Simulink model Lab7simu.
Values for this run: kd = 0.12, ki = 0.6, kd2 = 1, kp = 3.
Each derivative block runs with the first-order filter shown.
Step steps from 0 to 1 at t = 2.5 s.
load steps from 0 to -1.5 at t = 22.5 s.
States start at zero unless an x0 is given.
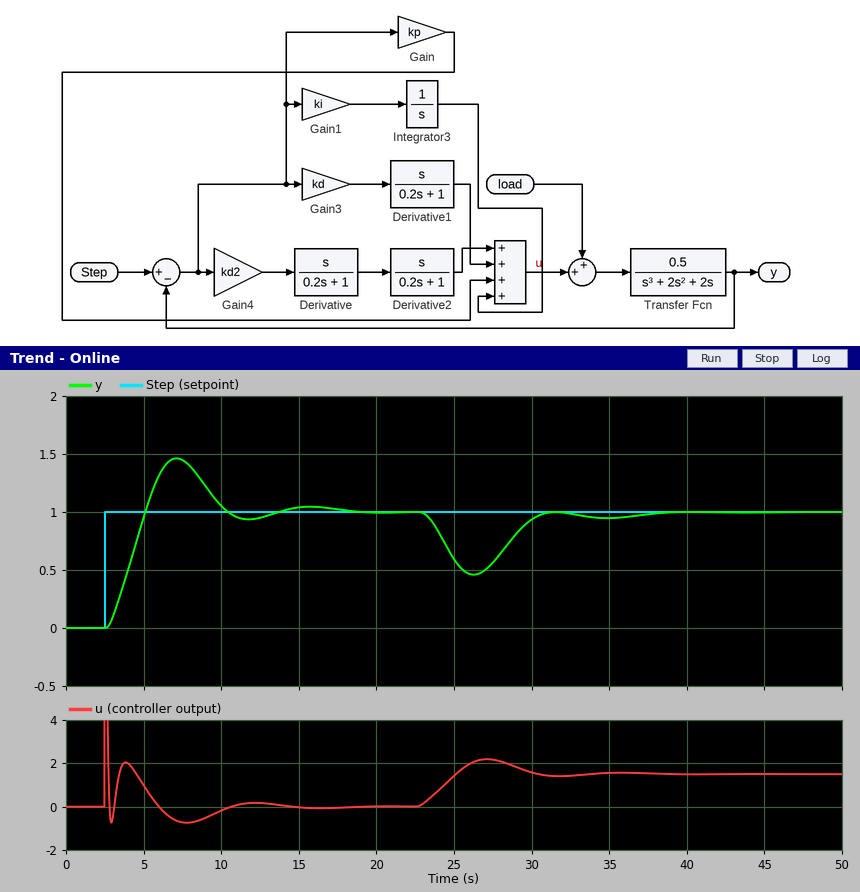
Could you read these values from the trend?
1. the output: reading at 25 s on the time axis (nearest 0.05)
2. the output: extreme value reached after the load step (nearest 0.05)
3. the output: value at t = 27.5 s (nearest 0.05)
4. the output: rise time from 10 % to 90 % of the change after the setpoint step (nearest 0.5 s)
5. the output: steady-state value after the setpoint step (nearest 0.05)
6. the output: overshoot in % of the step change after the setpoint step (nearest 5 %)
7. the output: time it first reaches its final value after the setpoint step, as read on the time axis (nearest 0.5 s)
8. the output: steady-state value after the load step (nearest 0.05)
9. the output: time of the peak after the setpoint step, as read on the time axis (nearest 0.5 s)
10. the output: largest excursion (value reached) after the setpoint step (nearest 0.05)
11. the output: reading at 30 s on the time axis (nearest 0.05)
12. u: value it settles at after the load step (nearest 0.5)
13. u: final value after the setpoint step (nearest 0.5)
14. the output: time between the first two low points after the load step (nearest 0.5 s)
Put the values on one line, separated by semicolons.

0.60; 0.45; 0.55; 2.0 s; 1.00; 45 %; 5.0 s; 1.00; 7.0 s; 1.45; 0.95; 1.5; 0.0; 8.5 s
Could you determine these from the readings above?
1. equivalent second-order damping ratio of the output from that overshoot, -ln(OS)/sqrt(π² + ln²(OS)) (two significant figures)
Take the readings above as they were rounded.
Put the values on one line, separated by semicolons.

0.25
